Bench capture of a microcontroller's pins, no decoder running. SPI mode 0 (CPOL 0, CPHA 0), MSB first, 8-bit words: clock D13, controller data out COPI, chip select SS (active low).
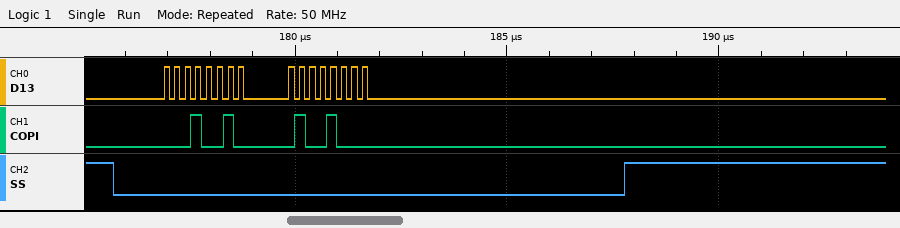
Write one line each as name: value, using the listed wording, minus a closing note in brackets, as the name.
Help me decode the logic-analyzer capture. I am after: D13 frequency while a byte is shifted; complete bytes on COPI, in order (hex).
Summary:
D13 frequency while a byte is shifted: 4 MHz
complete bytes on COPI, in order: 0x12 0x48
